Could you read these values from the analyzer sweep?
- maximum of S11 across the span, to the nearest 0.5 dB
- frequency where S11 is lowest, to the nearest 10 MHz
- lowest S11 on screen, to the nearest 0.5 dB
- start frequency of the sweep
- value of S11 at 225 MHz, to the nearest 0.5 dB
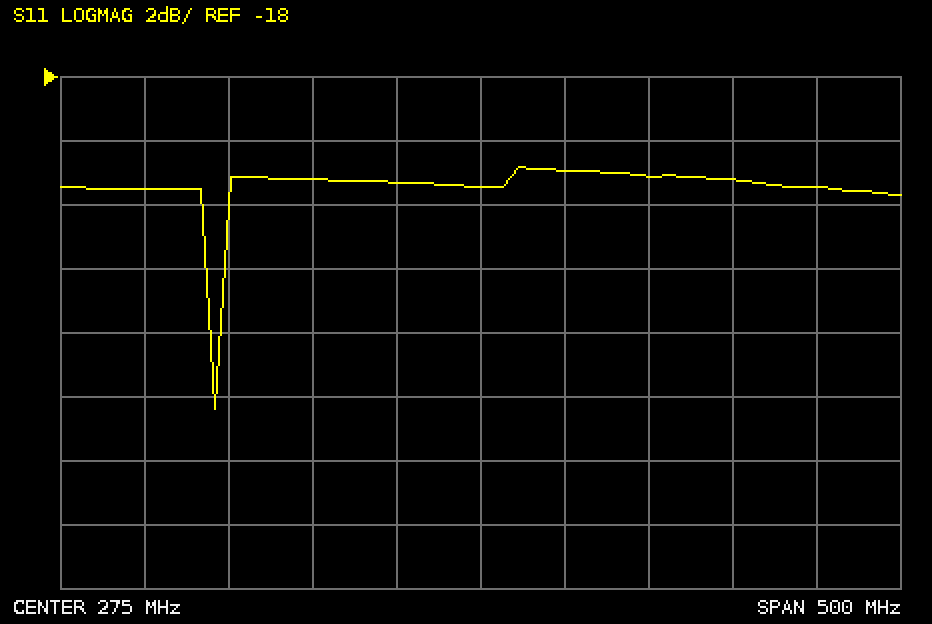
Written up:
-21.0 dB
120 MHz
-28.5 dB
25 MHz
-21.5 dB
